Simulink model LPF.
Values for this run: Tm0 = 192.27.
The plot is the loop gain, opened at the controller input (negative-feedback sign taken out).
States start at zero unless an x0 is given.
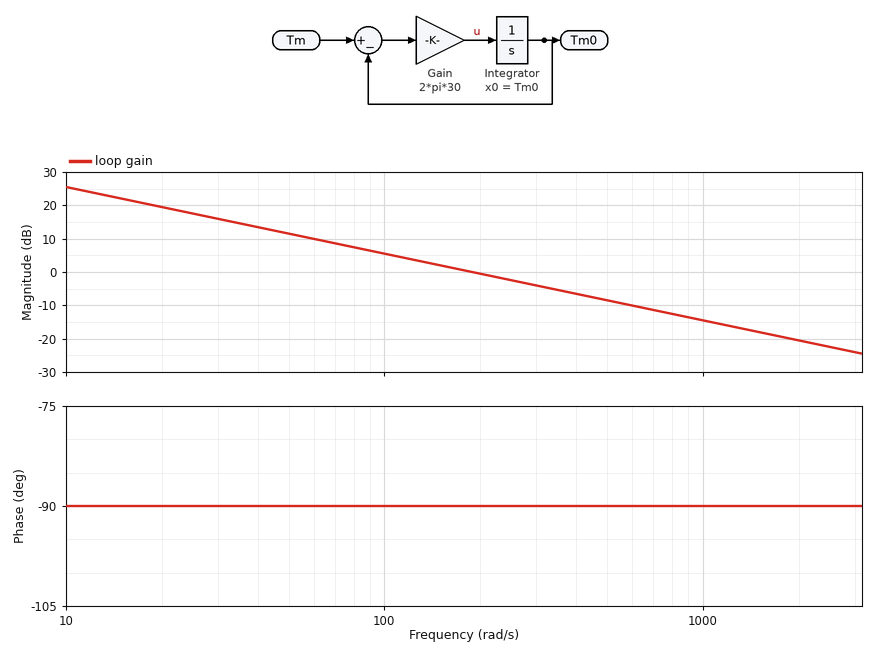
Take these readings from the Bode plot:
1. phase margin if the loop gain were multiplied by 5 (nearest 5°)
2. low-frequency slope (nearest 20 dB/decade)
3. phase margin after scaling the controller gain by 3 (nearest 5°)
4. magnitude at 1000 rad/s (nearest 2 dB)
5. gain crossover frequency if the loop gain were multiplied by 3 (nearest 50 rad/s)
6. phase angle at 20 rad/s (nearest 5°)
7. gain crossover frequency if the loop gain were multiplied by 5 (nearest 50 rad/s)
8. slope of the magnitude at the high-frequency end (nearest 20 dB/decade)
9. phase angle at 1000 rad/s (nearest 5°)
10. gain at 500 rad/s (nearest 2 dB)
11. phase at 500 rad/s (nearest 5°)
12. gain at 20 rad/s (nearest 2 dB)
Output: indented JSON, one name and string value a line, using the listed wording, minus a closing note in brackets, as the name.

{
  "phase margin if the loop gain were multiplied by 5": "90°",
  "low-frequency slope": "-20 dB/decade",
  "phase margin after scaling the controller gain by 3": "90°",
  "magnitude at 1000 rad/s": "-14 dB",
  "gain crossover frequency if the loop gain were multiplied by 3": "550 rad/s",
  "phase angle at 20 rad/s": "-90°",
  "gain crossover frequency if the loop gain were multiplied by 5": "950 rad/s",
  "slope of the magnitude at the high-frequency end": "-20 dB/decade",
  "phase angle at 1000 rad/s": "-90°",
  "gain at 500 rad/s": "-8 dB",
  "phase at 500 rad/s": "-90°",
  "gain at 20 rad/s": "20 dB"
}
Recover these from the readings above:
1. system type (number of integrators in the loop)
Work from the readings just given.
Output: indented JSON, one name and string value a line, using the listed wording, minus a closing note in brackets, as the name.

{
  "system type": "1"
}
